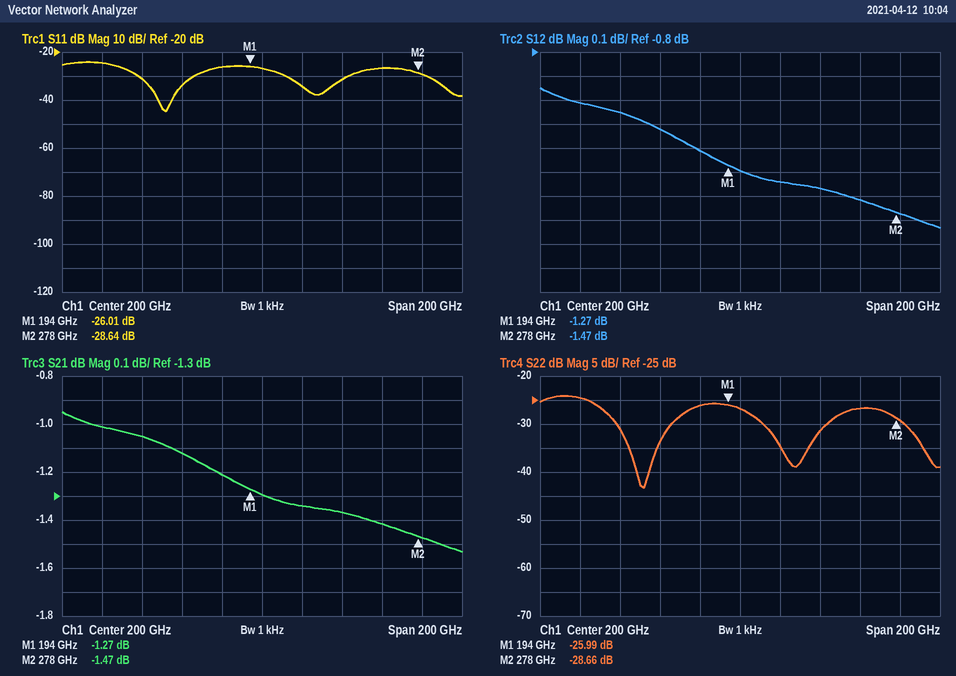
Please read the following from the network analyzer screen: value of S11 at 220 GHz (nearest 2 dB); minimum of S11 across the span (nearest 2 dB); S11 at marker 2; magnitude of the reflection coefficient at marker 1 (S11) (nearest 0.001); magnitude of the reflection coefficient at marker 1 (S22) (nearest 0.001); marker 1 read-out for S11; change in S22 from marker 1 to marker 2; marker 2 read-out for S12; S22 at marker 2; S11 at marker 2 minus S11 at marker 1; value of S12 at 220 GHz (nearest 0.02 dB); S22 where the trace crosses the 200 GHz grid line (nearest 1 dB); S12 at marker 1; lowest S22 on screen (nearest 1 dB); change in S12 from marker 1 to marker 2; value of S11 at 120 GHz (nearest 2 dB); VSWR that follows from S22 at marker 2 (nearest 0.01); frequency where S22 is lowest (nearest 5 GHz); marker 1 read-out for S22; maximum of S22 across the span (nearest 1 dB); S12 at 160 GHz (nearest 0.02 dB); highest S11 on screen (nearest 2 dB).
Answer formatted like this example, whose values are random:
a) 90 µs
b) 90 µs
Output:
a) -34 dB
b) -44 dB
c) -28.64 dB
d) 0.050
e) 0.050
f) -26.01 dB
g) -2.67 dB
h) -1.47 dB
i) -28.66 dB
j) -2.63 dB
k) -1.34 dB
l) -27 dB
m) -1.27 dB
n) -43 dB
o) -0.20 dB
p) -24 dB
q) 1.08
r) 150 GHz
s) -25.99 dB
t) -24 dB
u) -1.12 dB
v) -24 dB
